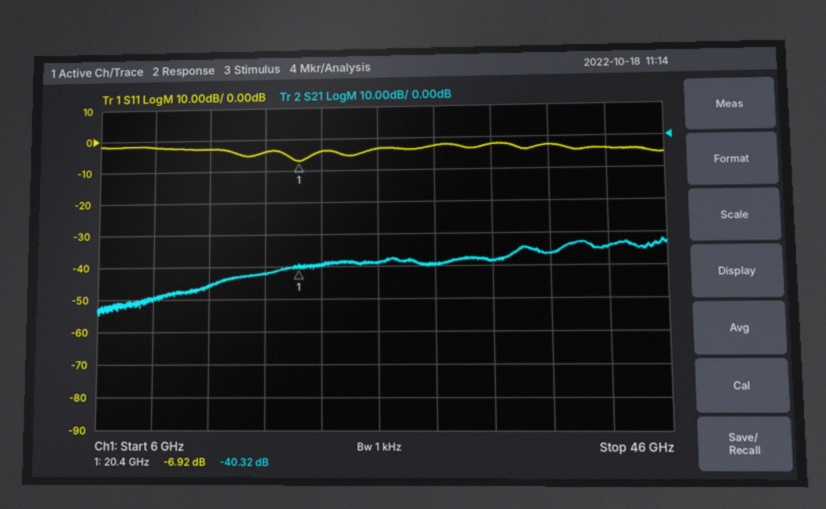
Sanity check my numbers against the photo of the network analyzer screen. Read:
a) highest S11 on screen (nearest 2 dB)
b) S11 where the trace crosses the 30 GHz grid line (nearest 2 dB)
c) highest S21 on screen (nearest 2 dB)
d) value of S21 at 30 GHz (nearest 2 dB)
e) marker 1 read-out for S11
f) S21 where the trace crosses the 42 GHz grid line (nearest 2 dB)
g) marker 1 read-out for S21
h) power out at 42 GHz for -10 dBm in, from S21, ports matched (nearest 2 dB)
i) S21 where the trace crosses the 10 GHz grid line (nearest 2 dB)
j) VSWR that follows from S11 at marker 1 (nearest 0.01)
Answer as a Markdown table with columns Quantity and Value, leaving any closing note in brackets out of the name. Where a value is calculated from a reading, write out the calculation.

| Quantity | Value |
|---|---|
| highest S11 on screen | -2 dB |
| S11 where the trace crosses the 30 GHz grid line | -2 dB |
| highest S21 on screen | -32 dB |
| value of S21 at 30 GHz | -40 dB |
| marker 1 read-out for S11 | -6.92 dB |
| S21 where the trace crosses the 42 GHz grid line | -34 dB |
| marker 1 read-out for S21 | -40.32 dB |
| power out at 42 GHz for -10 dBm in, from S21, ports matched | -10 dBm + (-34 dB) = -44 dBm |
| S21 where the trace crosses the 10 GHz grid line | -50 dB |
| VSWR that follows from S11 at marker 1 | (1 + 0.4508)/(1 − 0.4508) ≈ 2.64 |
